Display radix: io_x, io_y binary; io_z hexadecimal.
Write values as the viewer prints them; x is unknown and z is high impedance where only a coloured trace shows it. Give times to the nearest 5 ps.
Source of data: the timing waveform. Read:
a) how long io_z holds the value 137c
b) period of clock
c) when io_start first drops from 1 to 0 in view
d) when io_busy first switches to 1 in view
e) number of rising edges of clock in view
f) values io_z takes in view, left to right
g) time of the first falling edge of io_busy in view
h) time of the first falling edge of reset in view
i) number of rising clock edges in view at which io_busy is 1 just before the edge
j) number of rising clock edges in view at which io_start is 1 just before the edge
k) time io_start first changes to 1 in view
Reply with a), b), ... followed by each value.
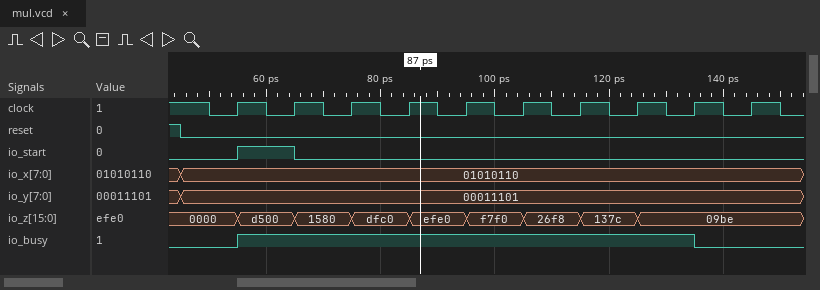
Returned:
a) 10 ps
b) 10 ps
c) 65 ps
d) 55 ps
e) 10
f) 0000, d500, 1580, dfc0, efe0, f7f0, 26f8, 137c, 09be
g) 135 ps
h) 45 ps
i) 8
j) 1
k) 55 ps
